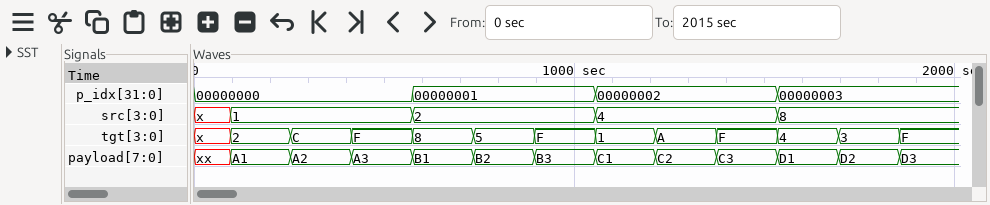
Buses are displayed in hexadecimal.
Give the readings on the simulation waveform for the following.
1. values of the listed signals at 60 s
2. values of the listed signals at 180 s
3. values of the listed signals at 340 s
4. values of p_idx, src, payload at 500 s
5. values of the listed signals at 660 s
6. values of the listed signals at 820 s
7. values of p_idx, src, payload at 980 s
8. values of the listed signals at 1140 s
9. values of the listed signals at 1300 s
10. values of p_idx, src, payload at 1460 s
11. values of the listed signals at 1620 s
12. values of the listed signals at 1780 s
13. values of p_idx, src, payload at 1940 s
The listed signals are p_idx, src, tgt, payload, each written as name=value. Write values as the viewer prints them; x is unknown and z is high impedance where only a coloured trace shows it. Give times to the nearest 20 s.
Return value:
p_idx=00000000, src=x, tgt=x, payload=xx
p_idx=00000000, src=1, tgt=2, payload=A1
p_idx=00000000, src=1, tgt=C, payload=A2
p_idx=00000000, src=1, payload=A3
p_idx=00000001, src=2, tgt=8, payload=B1
p_idx=00000001, src=2, tgt=5, payload=B2
p_idx=00000001, src=2, payload=B3
p_idx=00000002, src=4, tgt=1, payload=C1
p_idx=00000002, src=4, tgt=A, payload=C2
p_idx=00000002, src=4, payload=C3
p_idx=00000003, src=8, tgt=4, payload=D1
p_idx=00000003, src=8, tgt=3, payload=D2
p_idx=00000003, src=8, payload=D3
